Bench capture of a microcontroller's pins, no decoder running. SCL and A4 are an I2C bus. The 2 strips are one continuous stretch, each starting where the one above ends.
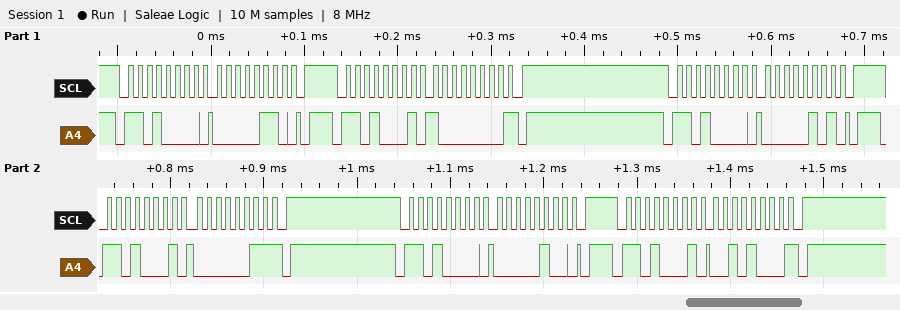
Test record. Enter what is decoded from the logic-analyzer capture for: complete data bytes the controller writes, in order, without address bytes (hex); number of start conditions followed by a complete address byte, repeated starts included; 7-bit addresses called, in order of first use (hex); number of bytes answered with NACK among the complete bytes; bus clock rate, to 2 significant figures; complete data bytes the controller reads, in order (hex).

06 05 04
6
0x68
3
100 kHz
80 03 28
